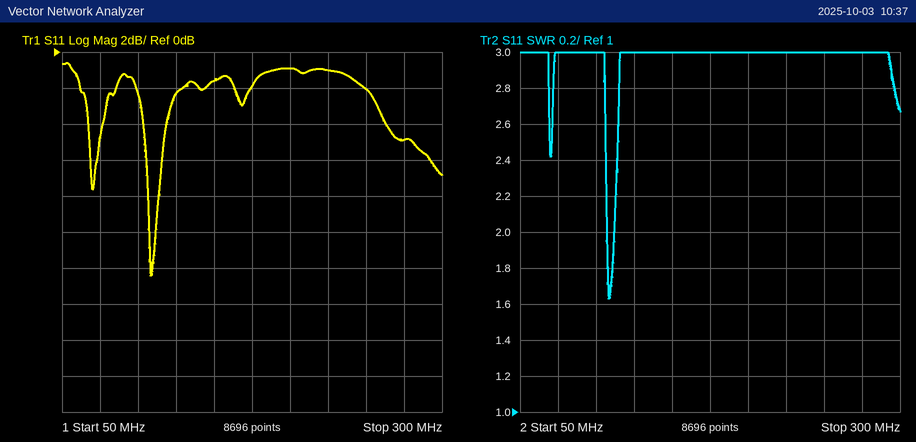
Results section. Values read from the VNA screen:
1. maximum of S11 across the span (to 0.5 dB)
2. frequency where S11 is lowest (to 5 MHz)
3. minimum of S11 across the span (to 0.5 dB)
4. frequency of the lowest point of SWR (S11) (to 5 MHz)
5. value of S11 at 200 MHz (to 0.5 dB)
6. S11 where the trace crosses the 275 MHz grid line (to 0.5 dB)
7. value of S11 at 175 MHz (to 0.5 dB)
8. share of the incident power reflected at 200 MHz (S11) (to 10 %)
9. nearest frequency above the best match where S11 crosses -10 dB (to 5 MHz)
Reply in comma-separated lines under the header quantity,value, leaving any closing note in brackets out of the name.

quantity,value
maximum of S11 across the span,-0.5 dB
frequency where S11 is lowest,110 MHz
minimum of S11 across the span,-12.5 dB
frequency of the lowest point of SWR (S11),110 MHz
value of S11 at 200 MHz,-1.0 dB
S11 where the trace crosses the 275 MHz grid line,-5.0 dB
value of S11 at 175 MHz,-2.0 dB
share of the incident power reflected at 200 MHz (S11),80 %
nearest frequency above the best match where S11 crosses -10 dB,110 MHz
